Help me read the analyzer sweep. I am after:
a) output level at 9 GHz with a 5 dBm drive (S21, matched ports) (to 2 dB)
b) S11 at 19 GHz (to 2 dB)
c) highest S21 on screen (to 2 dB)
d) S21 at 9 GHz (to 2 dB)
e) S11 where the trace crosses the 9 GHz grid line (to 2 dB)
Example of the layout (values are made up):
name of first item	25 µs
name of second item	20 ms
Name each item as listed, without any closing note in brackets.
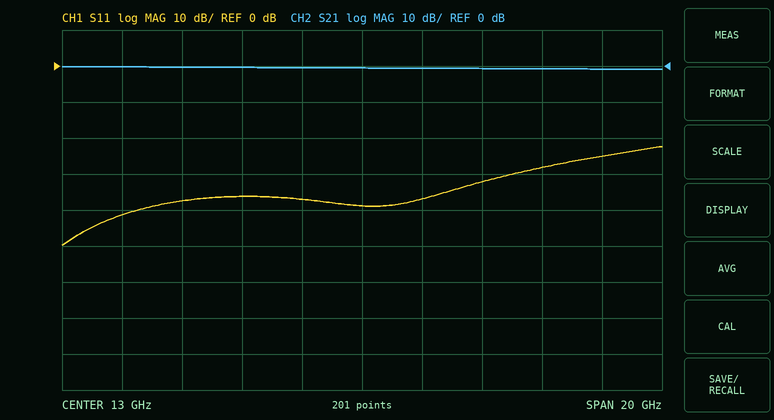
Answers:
output level at 9 GHz with a 5 dBm drive (S21, matched ports)	4 dBm
S11 at 19 GHz	-28 dB
highest S21 on screen	0 dB
S21 at 9 GHz	0 dB
S11 where the trace crosses the 9 GHz grid line	-36 dB
